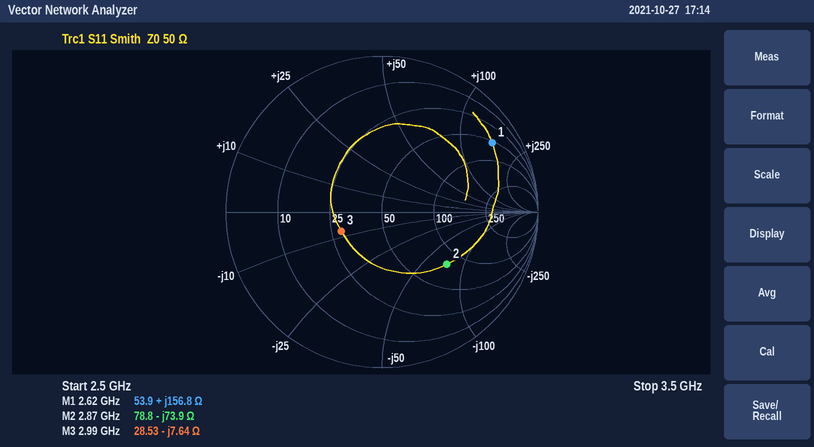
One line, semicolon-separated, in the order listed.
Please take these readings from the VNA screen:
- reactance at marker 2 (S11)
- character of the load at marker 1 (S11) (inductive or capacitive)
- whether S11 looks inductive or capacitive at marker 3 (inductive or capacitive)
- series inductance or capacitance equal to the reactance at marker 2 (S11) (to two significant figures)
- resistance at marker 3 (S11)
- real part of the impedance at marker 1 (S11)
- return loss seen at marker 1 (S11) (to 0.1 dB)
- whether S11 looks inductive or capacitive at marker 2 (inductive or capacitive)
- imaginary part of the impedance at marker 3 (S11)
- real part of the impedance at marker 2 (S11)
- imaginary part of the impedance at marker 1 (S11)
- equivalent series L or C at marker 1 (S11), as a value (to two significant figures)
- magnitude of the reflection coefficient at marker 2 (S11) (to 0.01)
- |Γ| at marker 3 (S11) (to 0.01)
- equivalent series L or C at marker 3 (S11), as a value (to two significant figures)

-73.9 Ω; inductive; capacitive; 750 fF; 28.53 Ω; 53.9 Ω; 1.6 dB; capacitive; -7.64 Ω; 78.8 Ω; +156.8 Ω; 9.5 nH; 0.53; 0.29; 7.0 pF
